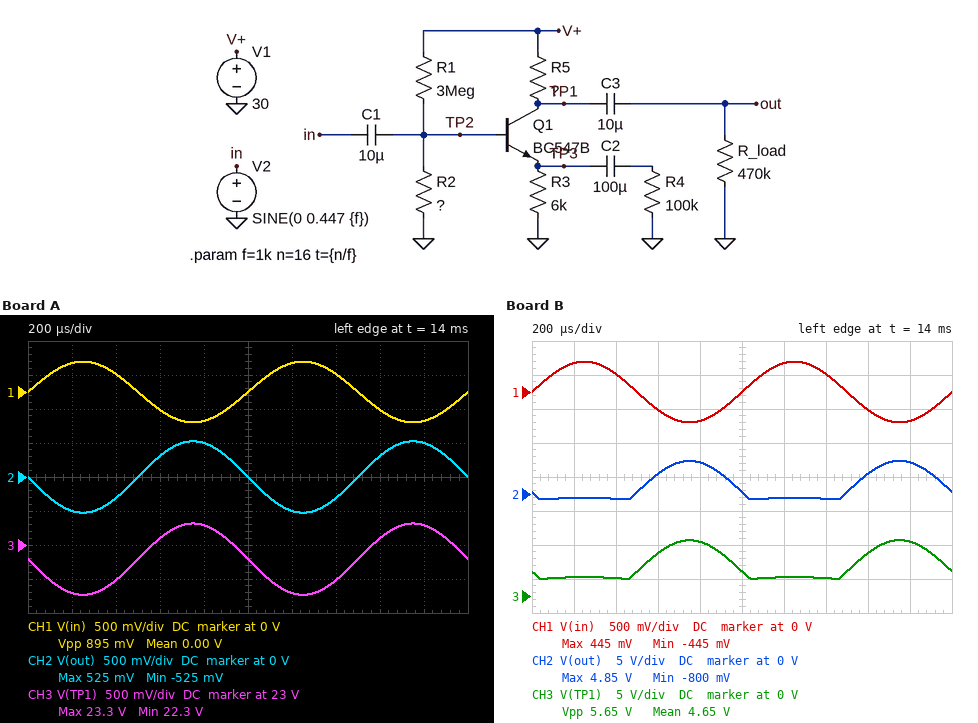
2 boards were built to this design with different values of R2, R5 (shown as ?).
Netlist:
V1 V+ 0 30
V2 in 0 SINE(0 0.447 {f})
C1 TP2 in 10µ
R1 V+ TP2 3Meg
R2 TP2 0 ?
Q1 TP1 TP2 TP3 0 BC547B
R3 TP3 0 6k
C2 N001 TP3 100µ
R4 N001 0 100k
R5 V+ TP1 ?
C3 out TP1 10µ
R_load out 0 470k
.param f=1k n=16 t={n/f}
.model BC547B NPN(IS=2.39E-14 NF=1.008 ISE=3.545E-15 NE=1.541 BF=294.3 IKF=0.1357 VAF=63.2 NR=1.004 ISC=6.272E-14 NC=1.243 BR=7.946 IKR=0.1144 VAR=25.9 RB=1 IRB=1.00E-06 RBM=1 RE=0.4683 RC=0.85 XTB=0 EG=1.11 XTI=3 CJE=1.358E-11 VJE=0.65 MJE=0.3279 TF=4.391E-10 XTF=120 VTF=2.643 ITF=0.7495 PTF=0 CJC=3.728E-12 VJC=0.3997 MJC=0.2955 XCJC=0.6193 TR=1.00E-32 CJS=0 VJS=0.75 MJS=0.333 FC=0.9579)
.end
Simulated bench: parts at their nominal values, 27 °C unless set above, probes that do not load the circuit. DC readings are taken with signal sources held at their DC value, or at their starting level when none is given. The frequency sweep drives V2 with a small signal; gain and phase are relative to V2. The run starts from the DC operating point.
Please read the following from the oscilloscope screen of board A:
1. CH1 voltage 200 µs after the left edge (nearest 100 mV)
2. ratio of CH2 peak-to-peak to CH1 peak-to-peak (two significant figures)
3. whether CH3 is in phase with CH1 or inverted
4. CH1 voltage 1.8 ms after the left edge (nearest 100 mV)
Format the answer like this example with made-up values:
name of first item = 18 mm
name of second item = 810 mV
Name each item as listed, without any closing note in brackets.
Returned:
CH1 voltage 200 µs after the left edge = 400 mV
ratio of CH2 peak-to-peak to CH1 peak-to-peak = 1.2
whether CH3 is in phase with CH1 or inverted = inverted
CH1 voltage 1.8 ms after the left edge = -400 mV
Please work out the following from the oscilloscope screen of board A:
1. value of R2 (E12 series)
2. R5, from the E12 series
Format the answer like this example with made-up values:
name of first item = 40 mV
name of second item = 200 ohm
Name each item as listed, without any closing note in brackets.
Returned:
value of R2 = 1.5 MΩ
R5, from the E12 series = 6.8 kΩ
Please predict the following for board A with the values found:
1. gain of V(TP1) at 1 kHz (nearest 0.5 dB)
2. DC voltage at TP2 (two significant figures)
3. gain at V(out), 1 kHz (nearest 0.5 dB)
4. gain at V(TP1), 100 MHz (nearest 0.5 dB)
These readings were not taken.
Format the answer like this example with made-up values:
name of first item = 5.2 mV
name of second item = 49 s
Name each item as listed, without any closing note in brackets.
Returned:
gain of V(TP1) at 1 kHz = 1.5 dB
DC voltage at TP2 = 7.0 V
gain at V(out), 1 kHz = 1.5 dB
gain at V(TP1), 100 MHz = 1.0 dB
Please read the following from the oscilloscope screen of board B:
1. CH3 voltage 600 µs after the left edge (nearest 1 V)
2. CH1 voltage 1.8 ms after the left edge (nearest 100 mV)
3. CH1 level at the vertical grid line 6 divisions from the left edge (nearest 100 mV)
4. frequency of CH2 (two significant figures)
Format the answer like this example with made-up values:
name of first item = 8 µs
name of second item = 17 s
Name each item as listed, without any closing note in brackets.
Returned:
CH3 voltage 600 µs after the left edge = 6 V
CH1 voltage 1.8 ms after the left edge = -400 mV
CH1 level at the vertical grid line 6 divisions from the left edge = 400 mV
frequency of CH2 = 1.0 kHz
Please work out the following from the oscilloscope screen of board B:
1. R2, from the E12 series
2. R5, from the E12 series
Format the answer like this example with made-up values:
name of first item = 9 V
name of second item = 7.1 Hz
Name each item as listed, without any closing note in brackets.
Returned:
R2, from the E12 series = 390 kΩ
R5, from the E12 series = 68 kΩ
